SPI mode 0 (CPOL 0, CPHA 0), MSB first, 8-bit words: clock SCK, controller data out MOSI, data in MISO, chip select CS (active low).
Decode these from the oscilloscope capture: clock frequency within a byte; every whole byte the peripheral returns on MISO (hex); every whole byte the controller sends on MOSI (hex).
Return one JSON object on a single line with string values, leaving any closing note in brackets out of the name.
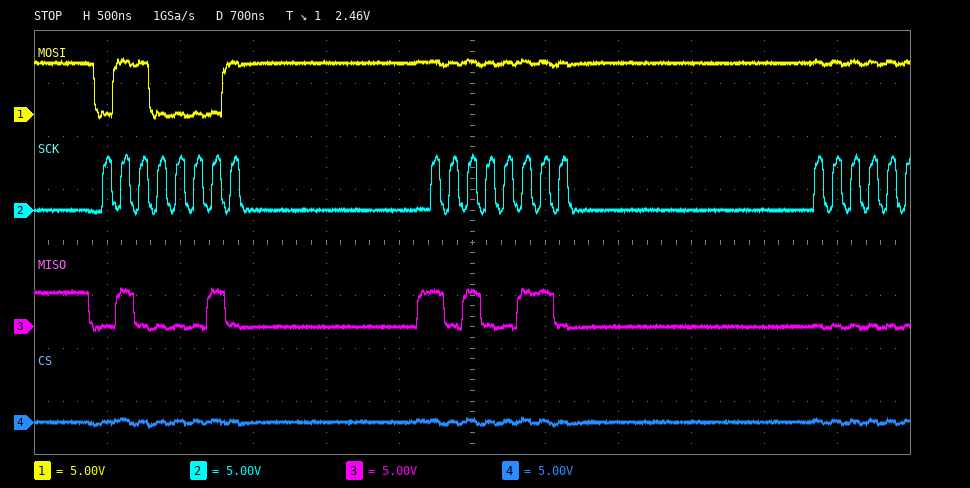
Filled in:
{"clock frequency within a byte": "8 MHz", "every whole byte the peripheral returns on MISO": "42 A6", "every whole byte the controller sends on MOSI": "61 FF"}
